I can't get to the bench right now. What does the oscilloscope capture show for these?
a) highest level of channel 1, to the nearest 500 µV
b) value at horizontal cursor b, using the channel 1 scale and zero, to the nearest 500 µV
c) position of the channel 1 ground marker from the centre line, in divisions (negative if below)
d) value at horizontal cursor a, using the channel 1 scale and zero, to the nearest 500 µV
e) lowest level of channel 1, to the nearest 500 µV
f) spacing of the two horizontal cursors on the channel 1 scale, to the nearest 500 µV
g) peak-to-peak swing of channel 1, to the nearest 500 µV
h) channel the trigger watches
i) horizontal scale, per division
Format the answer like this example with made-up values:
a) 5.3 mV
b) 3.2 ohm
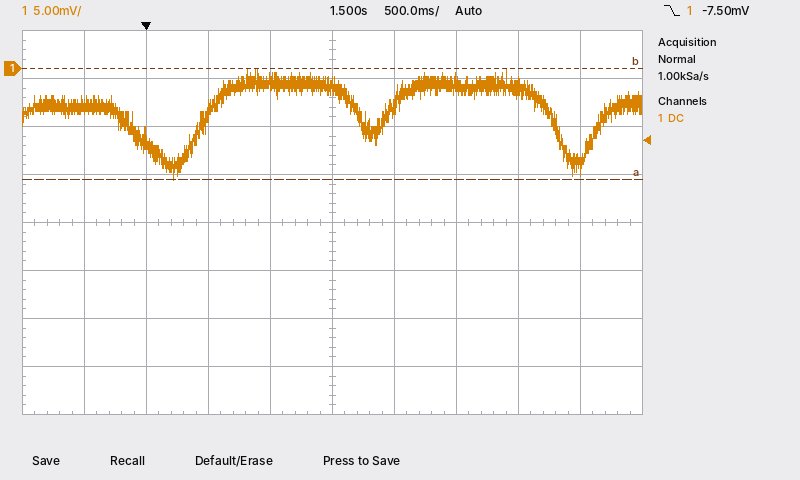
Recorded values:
a) 0.0 mV
b) 0.0 mV
c) +3.2 div
d) -11.5 mV
e) -11.5 mV
f) 11.5 mV
g) 11.5 mV
h) channel 1
i) 500 ms
